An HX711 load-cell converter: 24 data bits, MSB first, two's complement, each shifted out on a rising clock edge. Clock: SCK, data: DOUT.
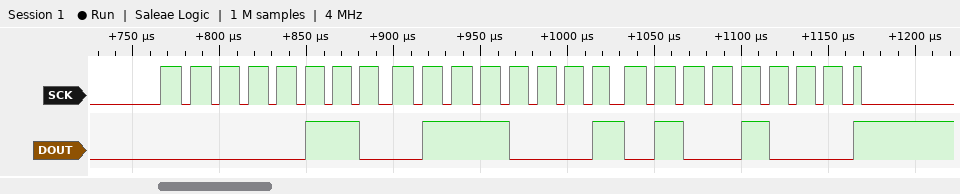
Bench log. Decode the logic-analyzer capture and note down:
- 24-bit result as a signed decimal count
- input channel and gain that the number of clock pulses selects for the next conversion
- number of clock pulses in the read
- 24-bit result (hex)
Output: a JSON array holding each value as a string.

["422216", "channel A, gain 128", "25", "0x067148"]
